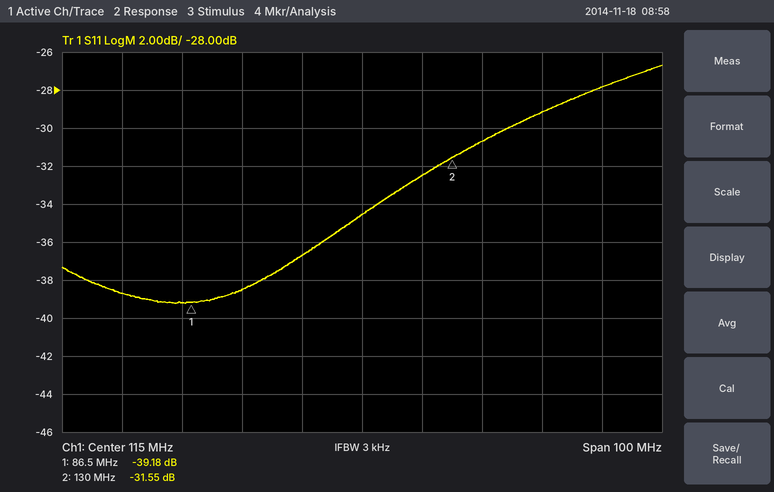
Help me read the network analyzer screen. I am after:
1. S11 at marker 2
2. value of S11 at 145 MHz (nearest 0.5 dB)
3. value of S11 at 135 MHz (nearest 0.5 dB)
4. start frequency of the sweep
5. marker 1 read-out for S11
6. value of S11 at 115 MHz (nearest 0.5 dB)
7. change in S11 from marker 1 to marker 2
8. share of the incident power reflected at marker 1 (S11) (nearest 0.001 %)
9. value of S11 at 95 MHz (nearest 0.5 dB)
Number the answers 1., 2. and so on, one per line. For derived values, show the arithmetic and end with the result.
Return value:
1. -31.55 dB
2. -29.0 dB
3. -30.5 dB
4. 65 MHz
5. -39.18 dB
6. -34.5 dB
7. -31.55 − (-39.18) = 7.63 dB
8. 10^(-39.18/10) ≈ 0.012 %
9. -38.5 dB
